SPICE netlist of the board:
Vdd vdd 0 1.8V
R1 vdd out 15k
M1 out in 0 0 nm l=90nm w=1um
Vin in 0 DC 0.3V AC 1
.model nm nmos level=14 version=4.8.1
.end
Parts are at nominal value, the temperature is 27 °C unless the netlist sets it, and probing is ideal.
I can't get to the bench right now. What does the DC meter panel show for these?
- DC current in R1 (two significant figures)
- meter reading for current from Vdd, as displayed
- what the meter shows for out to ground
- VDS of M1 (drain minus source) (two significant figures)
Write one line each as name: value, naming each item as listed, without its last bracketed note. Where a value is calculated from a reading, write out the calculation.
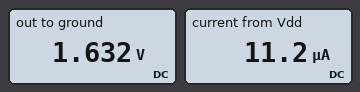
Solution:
DC current in R1: (1.8 V - 1.632 V) / 15 kΩ = 11 µA
meter reading for current from Vdd, as displayed: 11.2 µA
what the meter shows for out to ground: 1.632 V
VDS of M1 (drain minus source): 1.632 V = 1.6 V
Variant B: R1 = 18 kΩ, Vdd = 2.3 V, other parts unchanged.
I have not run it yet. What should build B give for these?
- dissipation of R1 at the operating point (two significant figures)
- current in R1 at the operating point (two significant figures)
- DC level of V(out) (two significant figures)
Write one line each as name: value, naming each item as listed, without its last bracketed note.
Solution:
dissipation of R1 at the operating point: 5.3 µW
current in R1 at the operating point: 17 µA
DC level of V(out): 2.0 V
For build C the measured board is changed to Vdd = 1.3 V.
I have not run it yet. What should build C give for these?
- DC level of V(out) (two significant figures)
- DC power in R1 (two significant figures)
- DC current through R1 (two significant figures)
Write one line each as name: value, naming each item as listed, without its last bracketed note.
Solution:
DC level of V(out): 1.2 V
DC power in R1: 670 nW
DC current through R1: 6.7 µA
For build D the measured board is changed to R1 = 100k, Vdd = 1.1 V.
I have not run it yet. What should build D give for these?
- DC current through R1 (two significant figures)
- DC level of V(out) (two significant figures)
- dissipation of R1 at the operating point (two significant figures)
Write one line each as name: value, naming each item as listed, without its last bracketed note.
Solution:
DC current through R1: 3.4 µA
DC level of V(out): 760 mV
dissipation of R1 at the operating point: 1.2 µW
